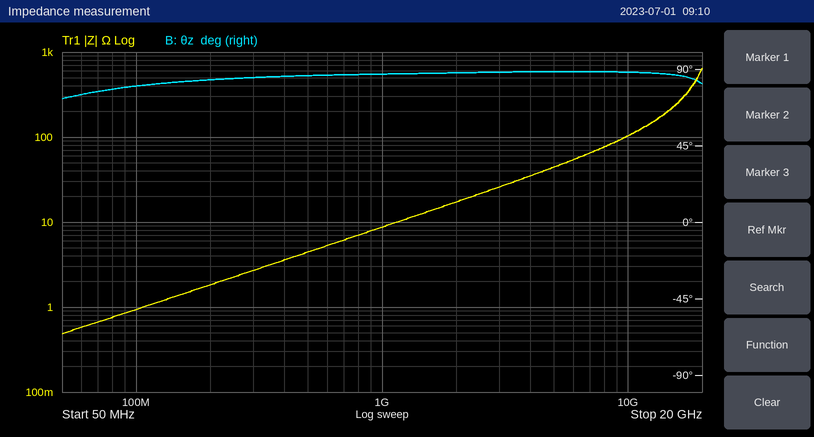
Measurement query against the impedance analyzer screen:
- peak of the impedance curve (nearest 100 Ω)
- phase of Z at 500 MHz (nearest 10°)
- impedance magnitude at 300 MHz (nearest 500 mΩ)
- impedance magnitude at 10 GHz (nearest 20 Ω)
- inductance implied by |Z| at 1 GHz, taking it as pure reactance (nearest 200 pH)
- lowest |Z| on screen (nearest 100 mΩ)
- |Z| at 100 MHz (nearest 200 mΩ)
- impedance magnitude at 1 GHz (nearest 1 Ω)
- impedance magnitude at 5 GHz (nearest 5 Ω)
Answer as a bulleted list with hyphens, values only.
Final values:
- 600 Ω
- 90°
- 2.5 Ω
- 100 Ω
- 1.4 nH
- 500 mΩ
- 1.0 Ω
- 9 Ω
- 45 Ω
